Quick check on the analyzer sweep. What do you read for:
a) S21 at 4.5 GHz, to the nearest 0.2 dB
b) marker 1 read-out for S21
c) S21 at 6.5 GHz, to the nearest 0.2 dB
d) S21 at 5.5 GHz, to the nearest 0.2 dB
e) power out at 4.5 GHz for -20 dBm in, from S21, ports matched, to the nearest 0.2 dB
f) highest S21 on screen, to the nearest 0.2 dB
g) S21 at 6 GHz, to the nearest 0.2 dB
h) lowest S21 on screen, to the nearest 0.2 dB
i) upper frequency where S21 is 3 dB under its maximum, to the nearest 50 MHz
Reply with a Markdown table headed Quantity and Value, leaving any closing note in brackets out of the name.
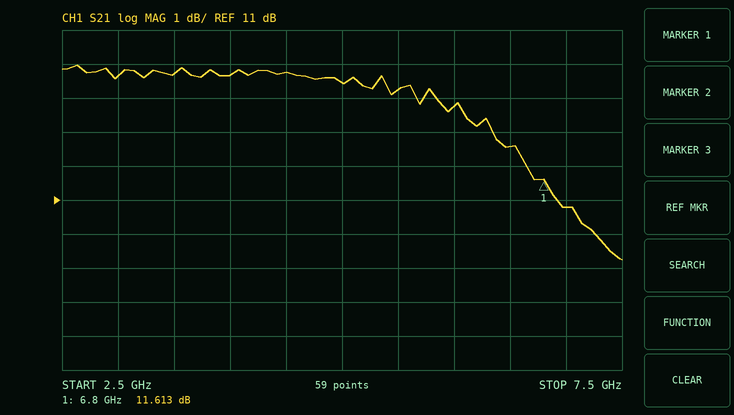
| Quantity | Value |
|---|---|
| S21 at 4.5 GHz, to the nearest 0.2 dB | 14.8 dB |
| marker 1 read-out for S21 | 11.613 dB |
| S21 at 6.5 GHz, to the nearest 0.2 dB | 12.6 dB |
| S21 at 5.5 GHz, to the nearest 0.2 dB | 14.2 dB |
| power out at 4.5 GHz for -20 dBm in, from S21, ports matched, to the nearest 0.2 dB | -5.2 dBm |
| highest S21 on screen, to the nearest 0.2 dB | 15.0 dB |
| S21 at 6 GHz, to the nearest 0.2 dB | 13.8 dB |
| lowest S21 on screen, to the nearest 0.2 dB | 9.2 dB |
| upper frequency where S21 is 3 dB under its maximum, to the nearest 50 MHz | 6.65 GHz |
